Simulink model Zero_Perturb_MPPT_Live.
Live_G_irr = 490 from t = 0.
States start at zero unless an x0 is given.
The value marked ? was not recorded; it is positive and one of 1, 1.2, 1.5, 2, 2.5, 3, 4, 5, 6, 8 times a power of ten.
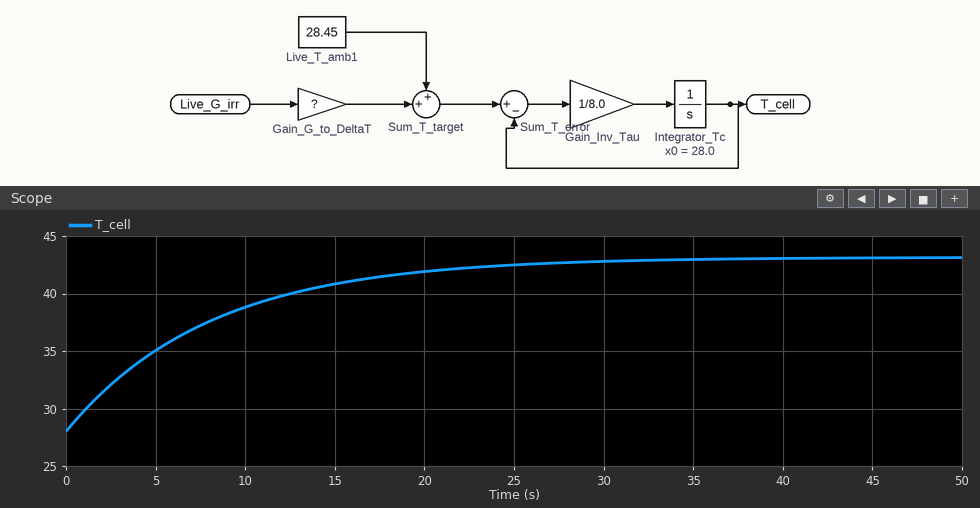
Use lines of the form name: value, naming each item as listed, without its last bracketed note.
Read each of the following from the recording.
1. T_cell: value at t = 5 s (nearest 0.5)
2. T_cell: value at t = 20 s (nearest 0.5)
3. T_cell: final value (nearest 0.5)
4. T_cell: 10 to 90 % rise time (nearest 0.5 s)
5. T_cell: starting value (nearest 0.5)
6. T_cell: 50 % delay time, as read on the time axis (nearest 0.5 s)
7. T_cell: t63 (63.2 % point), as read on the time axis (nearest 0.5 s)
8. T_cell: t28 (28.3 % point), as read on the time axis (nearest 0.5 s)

T_cell: value at t = 5 s: 35.0
T_cell: value at t = 20 s: 42.0
T_cell: final value: 43.0
T_cell: 10 to 90 % rise time: 17.5 s
T_cell: starting value: 28.0
T_cell: 50 % delay time, as read on the time axis: 5.5 s
T_cell: t63 (63.2 % point), as read on the time axis: 8.0 s
T_cell: t28 (28.3 % point), as read on the time axis: 2.5 s
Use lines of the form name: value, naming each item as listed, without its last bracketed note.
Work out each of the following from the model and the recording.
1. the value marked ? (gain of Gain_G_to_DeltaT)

the value marked ?: 0.03
